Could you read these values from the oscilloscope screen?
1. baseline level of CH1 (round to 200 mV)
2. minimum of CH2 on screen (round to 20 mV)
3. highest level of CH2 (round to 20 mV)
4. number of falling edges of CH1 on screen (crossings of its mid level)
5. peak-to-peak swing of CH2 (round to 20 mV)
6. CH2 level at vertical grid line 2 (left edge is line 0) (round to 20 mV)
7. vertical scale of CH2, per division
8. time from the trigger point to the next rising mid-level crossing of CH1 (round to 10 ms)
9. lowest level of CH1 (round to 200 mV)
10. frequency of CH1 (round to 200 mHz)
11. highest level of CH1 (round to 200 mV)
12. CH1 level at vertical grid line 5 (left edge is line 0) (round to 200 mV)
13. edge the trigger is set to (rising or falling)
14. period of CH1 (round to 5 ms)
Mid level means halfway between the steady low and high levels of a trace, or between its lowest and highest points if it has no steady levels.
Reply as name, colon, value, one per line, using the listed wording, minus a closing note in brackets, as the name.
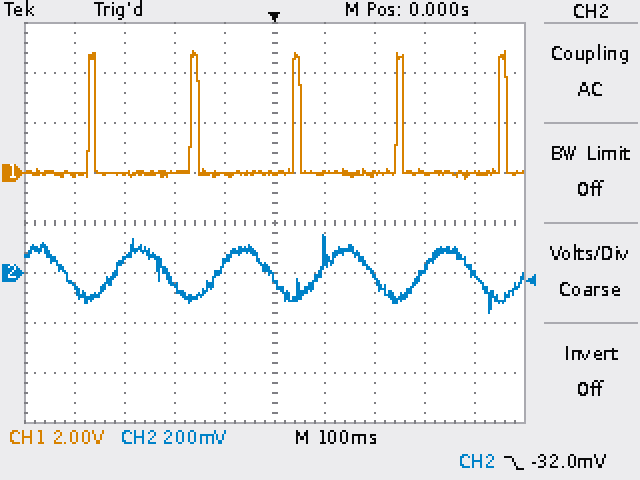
baseline level of CH1: 0.0 V
minimum of CH2 on screen: -160 mV
highest level of CH2: 160 mV
number of falling edges of CH1 on screen: 5
peak-to-peak swing of CH2: 320 mV
CH2 level at vertical grid line 2 (left edge is line 0): 60 mV
vertical scale of CH2, per division: 200 mV
time from the trigger point to the next rising mid-level crossing of CH1: 40 ms
lowest level of CH1: -200 mV
frequency of CH1: 4.8 Hz
highest level of CH1: 4.8 V
CH1 level at vertical grid line 5 (left edge is line 0): 0.0 V
edge the trigger is set to: falling
period of CH1: 205 ms
